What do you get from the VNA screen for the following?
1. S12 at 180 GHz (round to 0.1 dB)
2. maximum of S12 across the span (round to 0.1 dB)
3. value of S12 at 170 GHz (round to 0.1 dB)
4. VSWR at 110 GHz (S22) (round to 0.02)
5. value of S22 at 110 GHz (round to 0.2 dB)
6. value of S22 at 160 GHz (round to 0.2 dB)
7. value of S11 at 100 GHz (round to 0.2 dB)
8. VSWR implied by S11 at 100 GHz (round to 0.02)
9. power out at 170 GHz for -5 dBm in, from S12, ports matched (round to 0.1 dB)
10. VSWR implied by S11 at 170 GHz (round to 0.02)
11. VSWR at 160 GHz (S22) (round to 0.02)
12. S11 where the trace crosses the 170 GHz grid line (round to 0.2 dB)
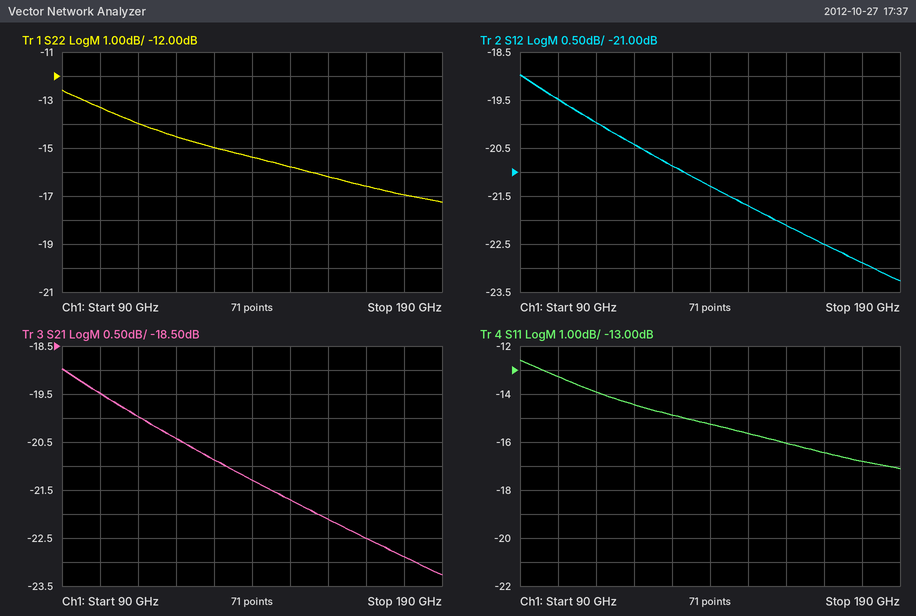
-22.9 dB
-19.0 dB
-22.5 dB
1.50
-14.0 dB
-16.2 dB
-13.2 dB
1.56
-27.5 dBm
1.36
1.36
-16.4 dB
